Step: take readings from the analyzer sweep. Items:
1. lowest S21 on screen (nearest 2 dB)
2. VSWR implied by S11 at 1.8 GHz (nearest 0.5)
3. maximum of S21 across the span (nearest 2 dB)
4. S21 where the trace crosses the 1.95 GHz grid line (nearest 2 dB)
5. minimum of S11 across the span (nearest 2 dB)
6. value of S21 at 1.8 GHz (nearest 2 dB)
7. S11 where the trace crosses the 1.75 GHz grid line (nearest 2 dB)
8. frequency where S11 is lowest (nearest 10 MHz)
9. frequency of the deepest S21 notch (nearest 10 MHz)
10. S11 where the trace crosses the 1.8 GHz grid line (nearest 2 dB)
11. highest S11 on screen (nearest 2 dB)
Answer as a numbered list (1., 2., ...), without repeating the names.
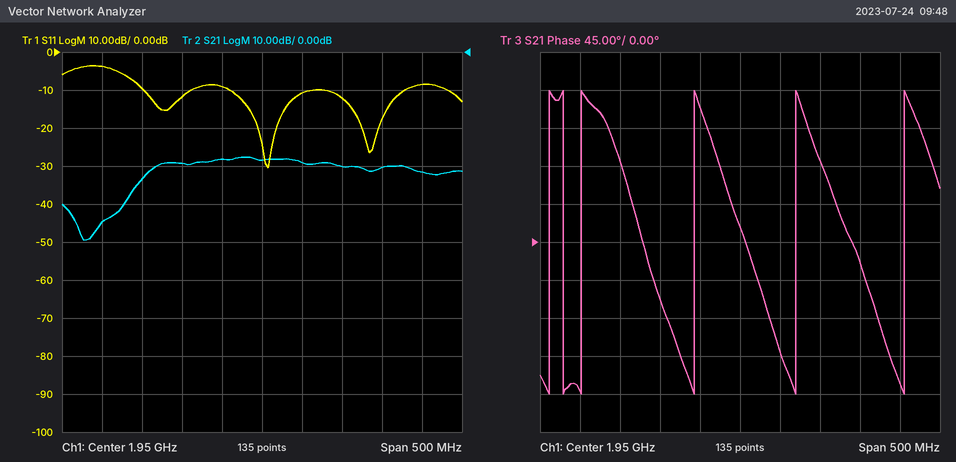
1. -50 dB
2. 2.0
3. -28 dB
4. -28 dB
5. -30 dB
6. -34 dB
7. -4 dB
8. 1.96 GHz
9. 1.73 GHz
10. -10 dB
11. -4 dB
